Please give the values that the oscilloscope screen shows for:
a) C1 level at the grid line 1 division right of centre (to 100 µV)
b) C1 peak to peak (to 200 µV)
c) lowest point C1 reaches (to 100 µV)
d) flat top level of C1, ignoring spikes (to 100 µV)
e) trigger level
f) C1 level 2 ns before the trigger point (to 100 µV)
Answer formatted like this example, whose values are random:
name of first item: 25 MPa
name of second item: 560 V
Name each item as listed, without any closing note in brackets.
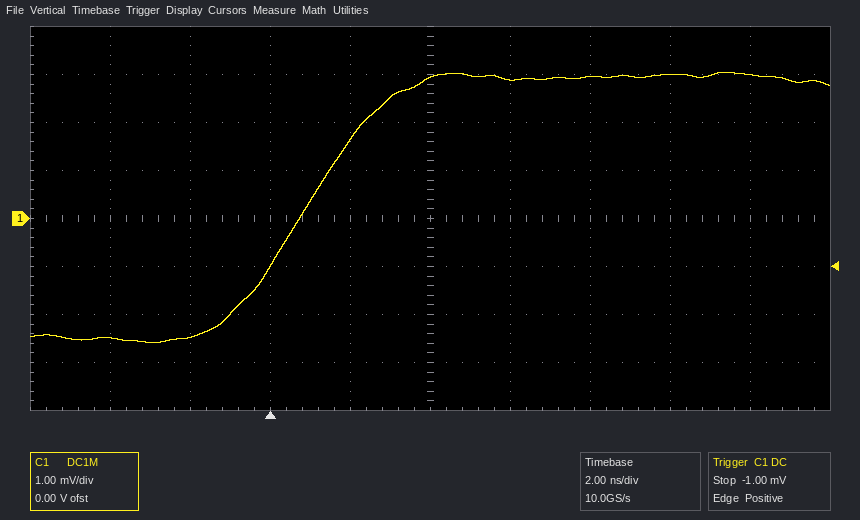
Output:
C1 level at the grid line 1 division right of centre: 2.9 mV
C1 peak to peak: 5.6 mV
lowest point C1 reaches: -2.6 mV
flat top level of C1, ignoring spikes: 3.0 mV
trigger level: -1.00 mV
C1 level 2 ns before the trigger point: -2.5 mV
